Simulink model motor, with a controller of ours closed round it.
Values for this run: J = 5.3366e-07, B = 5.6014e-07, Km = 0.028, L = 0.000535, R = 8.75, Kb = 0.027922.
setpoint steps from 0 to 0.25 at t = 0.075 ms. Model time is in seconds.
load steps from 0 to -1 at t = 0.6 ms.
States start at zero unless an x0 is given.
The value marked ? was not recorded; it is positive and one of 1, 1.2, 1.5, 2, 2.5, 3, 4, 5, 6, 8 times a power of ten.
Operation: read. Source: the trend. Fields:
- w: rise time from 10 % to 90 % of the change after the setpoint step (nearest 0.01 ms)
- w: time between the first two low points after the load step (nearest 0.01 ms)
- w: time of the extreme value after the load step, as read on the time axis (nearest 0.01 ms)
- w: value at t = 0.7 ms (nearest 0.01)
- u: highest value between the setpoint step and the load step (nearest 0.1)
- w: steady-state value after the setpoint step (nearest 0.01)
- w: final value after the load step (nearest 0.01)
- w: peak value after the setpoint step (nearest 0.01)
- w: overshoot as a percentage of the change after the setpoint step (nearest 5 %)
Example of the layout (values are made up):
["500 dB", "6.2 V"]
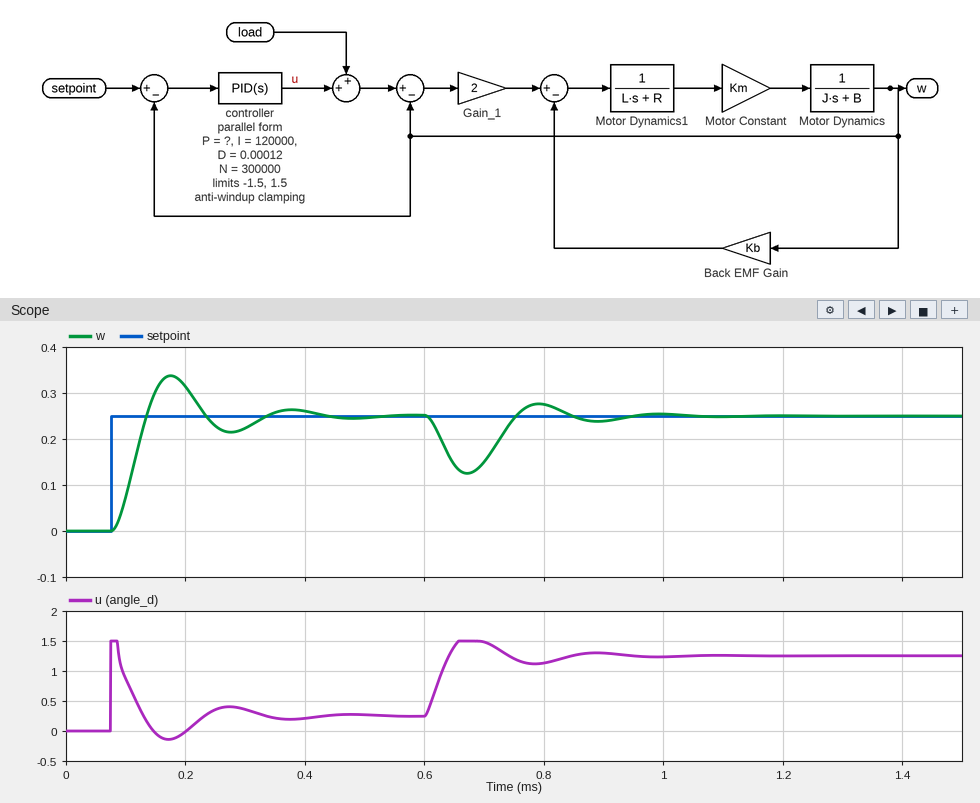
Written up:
["0.04 ms", "0.22 ms", "0.67 ms", "0.15", "1.5", "0.25", "0.25", "0.34", "35 %"]
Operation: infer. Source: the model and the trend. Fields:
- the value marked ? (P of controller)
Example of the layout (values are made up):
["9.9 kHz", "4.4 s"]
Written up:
["6"]
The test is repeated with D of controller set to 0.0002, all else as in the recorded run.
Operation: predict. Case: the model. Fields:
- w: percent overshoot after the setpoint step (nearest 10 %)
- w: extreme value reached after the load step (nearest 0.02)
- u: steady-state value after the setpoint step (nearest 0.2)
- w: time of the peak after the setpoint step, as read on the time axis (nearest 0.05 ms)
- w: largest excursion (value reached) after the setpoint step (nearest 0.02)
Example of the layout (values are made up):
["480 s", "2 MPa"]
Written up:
["30 %", "0.14", "0.2", "0.20 ms", "0.32"]
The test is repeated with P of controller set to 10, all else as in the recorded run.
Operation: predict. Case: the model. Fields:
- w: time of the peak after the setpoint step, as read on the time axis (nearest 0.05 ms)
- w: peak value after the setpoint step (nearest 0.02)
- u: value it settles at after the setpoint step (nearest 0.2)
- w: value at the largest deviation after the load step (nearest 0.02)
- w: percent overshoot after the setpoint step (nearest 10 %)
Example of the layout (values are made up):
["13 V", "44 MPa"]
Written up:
["0.15 ms", "0.30", "0.2", "0.16", "20 %"]
